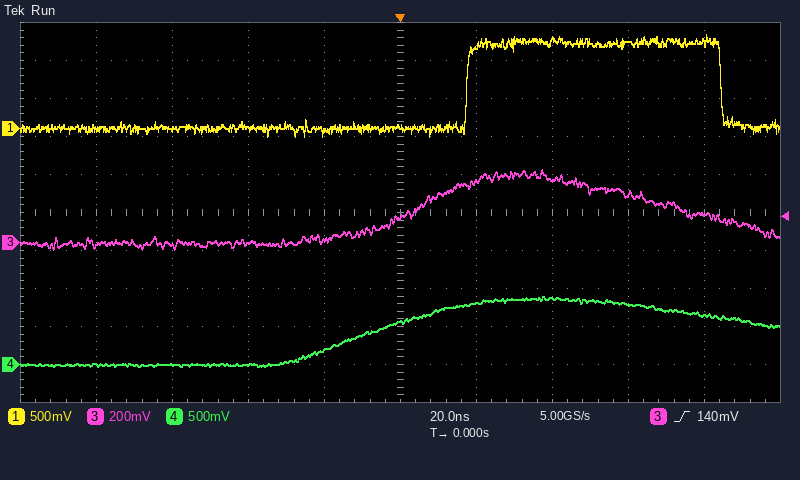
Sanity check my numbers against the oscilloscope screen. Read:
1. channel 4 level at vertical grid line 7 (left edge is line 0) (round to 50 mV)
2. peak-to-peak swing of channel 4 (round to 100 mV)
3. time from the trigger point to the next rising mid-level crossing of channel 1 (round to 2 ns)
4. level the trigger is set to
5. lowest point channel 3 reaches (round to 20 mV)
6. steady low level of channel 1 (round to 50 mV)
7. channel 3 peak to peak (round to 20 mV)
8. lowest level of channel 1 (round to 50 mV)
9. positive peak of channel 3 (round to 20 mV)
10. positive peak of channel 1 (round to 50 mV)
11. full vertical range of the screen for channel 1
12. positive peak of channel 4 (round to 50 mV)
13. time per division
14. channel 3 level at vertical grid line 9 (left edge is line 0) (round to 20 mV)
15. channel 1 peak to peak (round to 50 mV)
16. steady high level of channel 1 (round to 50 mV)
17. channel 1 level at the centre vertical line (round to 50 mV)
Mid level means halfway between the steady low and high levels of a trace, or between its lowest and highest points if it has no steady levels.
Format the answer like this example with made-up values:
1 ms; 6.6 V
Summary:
850 mV; 900 mV; 18 ns; 140 mV; -40 mV; 0 mV; 420 mV; -100 mV; 380 mV; 1.25 V; 5 V; 900 mV; 20 ns; 160 mV; 1.35 V; 1.15 V; 0 mV
